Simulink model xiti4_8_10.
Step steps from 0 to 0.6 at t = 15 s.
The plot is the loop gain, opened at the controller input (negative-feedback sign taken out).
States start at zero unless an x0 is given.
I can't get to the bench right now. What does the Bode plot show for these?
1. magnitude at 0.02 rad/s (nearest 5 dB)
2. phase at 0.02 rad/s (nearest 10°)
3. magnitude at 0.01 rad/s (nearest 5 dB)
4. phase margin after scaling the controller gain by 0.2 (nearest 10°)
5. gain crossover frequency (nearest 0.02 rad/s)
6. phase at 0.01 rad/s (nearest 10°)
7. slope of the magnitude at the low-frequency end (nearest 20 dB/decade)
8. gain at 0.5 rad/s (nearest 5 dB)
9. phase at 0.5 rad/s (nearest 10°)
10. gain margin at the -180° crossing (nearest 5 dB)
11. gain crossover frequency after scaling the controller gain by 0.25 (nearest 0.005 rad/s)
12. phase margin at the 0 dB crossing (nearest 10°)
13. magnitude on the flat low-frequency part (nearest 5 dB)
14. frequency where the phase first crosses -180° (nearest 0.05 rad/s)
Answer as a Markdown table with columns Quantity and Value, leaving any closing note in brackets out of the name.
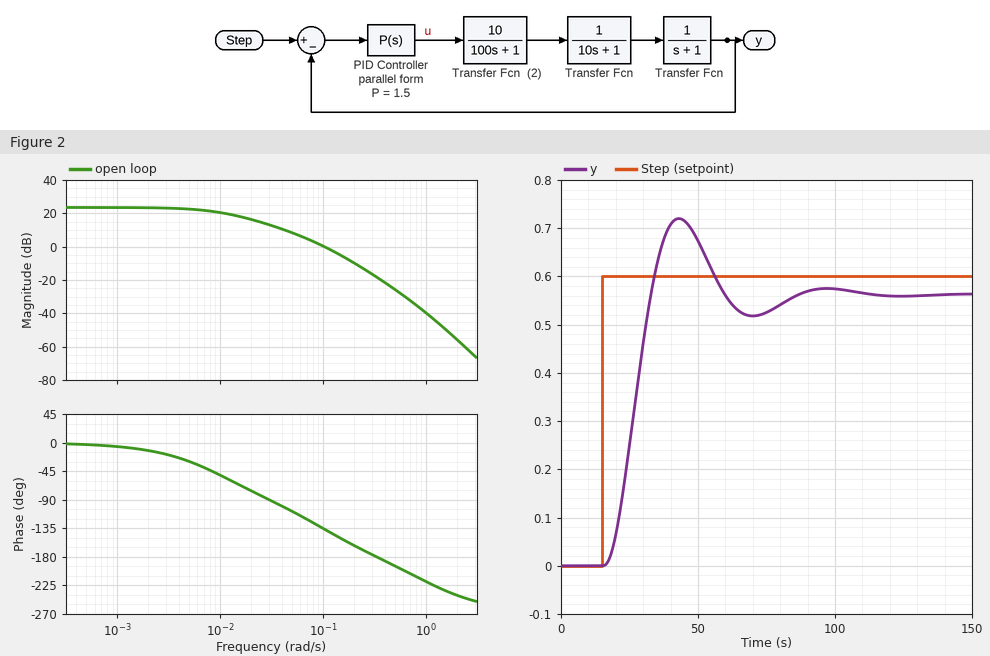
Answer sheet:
| Quantity | Value |
|---|---|
| magnitude at 0.02 rad/s | 15 dB |
| phase at 0.02 rad/s | -80° |
| magnitude at 0.01 rad/s | 20 dB |
| phase margin after scaling the controller gain by 0.2 | 90° |
| gain crossover frequency | 0.10 rad/s |
| phase at 0.01 rad/s | -50° |
| slope of the magnitude at the low-frequency end | 0 dB/decade |
| gain at 0.5 rad/s | -25 dB |
| phase at 0.5 rad/s | -190° |
| gain margin at the -180° crossing | 20 dB |
| gain crossover frequency after scaling the controller gain by 0.25 | 0.035 rad/s |
| phase margin at the 0 dB crossing | 40° |
| magnitude on the flat low-frequency part | 25 dB |
| frequency where the phase first crosses -180° | 0.35 rad/s |
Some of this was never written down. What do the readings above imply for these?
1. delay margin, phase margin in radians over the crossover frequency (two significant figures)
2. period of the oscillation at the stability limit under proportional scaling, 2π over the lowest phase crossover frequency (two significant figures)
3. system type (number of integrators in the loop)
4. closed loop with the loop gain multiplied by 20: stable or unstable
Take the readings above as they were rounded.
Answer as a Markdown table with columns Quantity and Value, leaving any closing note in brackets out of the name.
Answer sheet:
| Quantity | Value |
|---|---|
| delay margin, phase margin in radians over the crossover frequency | 7.0 s |
| period of the oscillation at the stability limit under proportional scaling, 2π over the lowest phase crossover frequency | 18 s |
| system type | 0 |
| closed loop with the loop gain multiplied by 20: stable or unstable | unstable |
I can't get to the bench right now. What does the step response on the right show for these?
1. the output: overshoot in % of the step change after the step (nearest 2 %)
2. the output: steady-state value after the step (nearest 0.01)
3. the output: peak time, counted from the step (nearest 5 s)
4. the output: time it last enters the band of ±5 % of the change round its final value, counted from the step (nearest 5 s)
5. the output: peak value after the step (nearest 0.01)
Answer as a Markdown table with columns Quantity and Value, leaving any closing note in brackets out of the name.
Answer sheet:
| Quantity | Value |
|---|---|
| the output: overshoot in % of the step change after the step | 28 % |
| the output: steady-state value after the step | 0.56 |
| the output: peak time, counted from the step | 30 s |
| the output: time it last enters the band of ±5 % of the change round its final value, counted from the step | 65 s |
| the output: peak value after the step | 0.72 |
